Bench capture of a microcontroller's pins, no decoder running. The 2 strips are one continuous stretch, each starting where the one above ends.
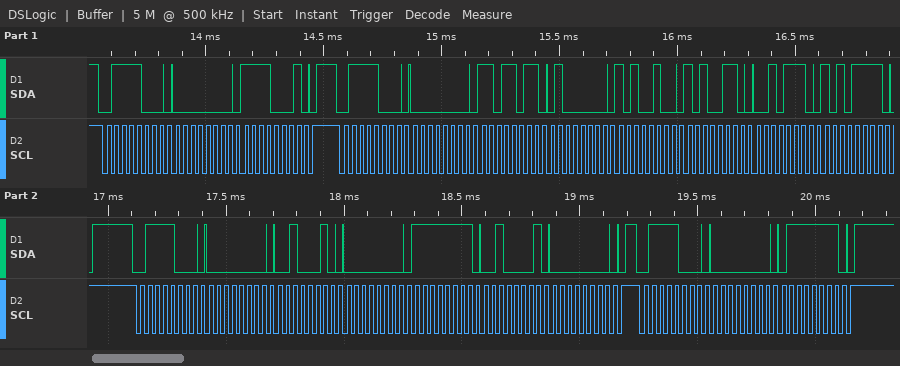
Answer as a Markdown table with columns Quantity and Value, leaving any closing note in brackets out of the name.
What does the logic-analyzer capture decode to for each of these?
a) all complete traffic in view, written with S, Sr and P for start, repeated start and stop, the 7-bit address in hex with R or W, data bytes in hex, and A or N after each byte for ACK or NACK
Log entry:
| Quantity | Value |
|---|---|
| all complete traffic in view, written with S, Sr and P for start, repeated start and stop, the 7-bit address in hex with R or W, data bytes in hex, and A or N after each byte for ACK or NACK | S 3CW A 00 A F1 A P S 3CW A 00 A DB A 40 A A4 A A6 A 2E A AF A P S 3CW A 00 A 22 A 00 A FF A 21 A 00 A P S 3CW A 00 A 7F A P |
